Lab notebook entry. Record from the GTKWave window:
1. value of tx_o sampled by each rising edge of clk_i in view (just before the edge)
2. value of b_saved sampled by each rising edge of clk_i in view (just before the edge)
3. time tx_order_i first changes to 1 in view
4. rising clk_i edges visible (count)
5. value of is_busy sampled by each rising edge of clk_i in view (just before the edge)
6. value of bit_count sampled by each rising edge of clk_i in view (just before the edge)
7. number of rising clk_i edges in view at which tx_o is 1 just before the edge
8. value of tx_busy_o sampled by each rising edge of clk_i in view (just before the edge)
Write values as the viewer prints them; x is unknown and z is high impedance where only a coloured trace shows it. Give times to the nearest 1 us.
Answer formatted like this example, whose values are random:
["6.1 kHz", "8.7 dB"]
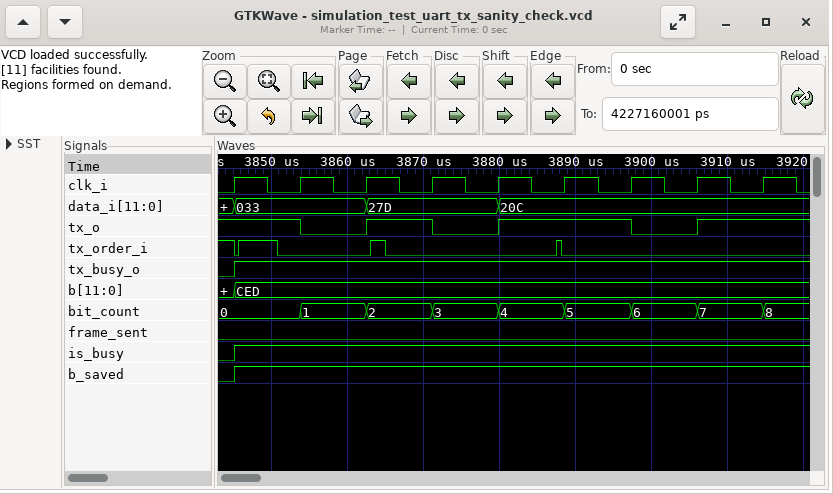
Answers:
["1 1 0 1 0 1 1 0 1", "0 1 1 1 1 1 1 1 1", "3846 us", "9", "0 1 1 1 1 1 1 1 1", "0, 0, 1, 2, 3, 4, 5, 6, 7", "6", "0 1 1 1 1 1 1 1 1"]
